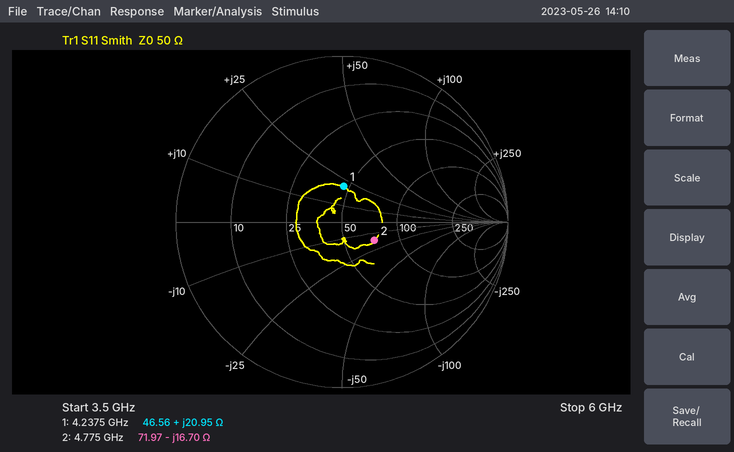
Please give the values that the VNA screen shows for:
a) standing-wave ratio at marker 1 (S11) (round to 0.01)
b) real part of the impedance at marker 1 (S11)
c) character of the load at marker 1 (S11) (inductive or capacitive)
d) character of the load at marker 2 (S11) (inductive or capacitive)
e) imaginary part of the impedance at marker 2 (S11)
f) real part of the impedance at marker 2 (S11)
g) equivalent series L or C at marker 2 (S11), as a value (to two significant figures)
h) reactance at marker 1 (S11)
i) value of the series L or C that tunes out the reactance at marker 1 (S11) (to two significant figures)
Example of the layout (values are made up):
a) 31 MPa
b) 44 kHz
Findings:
a) 1.55
b) 46.56 Ω
c) inductive
d) capacitive
e) -16.70 Ω
f) 71.97 Ω
g) 2.0 pF
h) +20.95 Ω
i) 1.8 pF
